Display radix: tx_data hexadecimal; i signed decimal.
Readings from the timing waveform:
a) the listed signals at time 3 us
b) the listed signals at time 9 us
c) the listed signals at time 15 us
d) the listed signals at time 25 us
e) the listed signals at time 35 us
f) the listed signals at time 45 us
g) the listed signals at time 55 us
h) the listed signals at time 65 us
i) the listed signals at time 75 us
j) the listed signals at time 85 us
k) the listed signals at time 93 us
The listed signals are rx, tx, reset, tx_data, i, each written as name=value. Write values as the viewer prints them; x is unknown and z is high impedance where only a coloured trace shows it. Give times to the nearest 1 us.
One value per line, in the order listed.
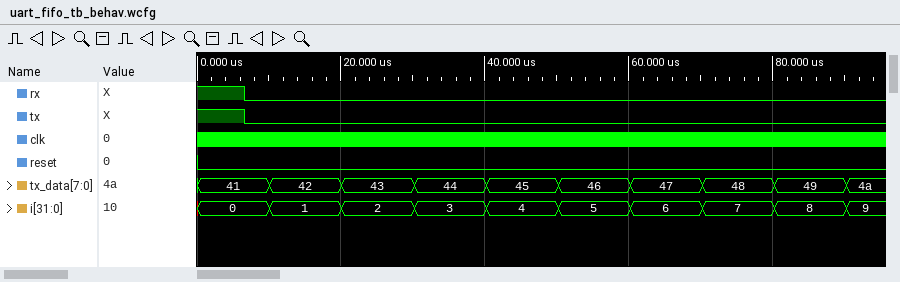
rx=1, tx=1, reset=0, tx_data=41, i=0
rx=0, tx=0, reset=0, tx_data=41, i=0
rx=0, tx=0, reset=0, tx_data=42, i=1
rx=0, tx=0, reset=0, tx_data=43, i=2
rx=0, tx=0, reset=0, tx_data=44, i=3
rx=0, tx=0, reset=0, tx_data=45, i=4
rx=0, tx=0, reset=0, tx_data=46, i=5
rx=0, tx=0, reset=0, tx_data=47, i=6
rx=0, tx=0, reset=0, tx_data=48, i=7
rx=0, tx=0, reset=0, tx_data=49, i=8
rx=0, tx=0, reset=0, tx_data=4a, i=9
